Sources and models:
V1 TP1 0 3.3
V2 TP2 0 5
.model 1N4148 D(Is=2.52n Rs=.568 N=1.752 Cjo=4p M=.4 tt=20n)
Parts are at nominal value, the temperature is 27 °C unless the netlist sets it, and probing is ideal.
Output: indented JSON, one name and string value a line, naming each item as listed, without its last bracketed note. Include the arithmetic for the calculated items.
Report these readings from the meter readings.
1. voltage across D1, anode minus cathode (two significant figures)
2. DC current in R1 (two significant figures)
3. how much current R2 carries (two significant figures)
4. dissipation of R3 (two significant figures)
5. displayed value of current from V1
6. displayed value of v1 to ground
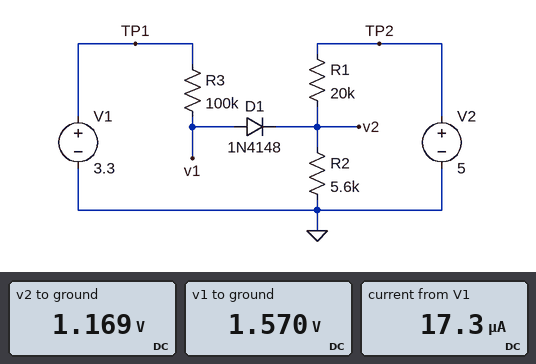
{
  "voltage across D1, anode minus cathode": "1.57 V - 1.169 V = 400 mV",
  "DC current in R1": "(5 V - 1.169 V) / 20 kΩ = 190 µA",
  "how much current R2 carries": "(1.169 V) / 5.6 kΩ = 210 µA",
  "dissipation of R3": "(3.3 V - 1.57 V)^2 / 100 kΩ = 30 µW",
  "displayed value of current from V1": "17.3 µA",
  "displayed value of v1 to ground": "1.570 V"
}
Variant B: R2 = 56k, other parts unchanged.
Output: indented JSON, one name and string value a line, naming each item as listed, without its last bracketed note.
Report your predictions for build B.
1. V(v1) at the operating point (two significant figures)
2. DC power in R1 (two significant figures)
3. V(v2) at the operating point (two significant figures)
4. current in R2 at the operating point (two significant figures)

{
  "V(v1) at the operating point": "3.3 V",
  "DC power in R1": "87 µW",
  "V(v2) at the operating point": "3.7 V",
  "current in R2 at the operating point": "66 µA"
}
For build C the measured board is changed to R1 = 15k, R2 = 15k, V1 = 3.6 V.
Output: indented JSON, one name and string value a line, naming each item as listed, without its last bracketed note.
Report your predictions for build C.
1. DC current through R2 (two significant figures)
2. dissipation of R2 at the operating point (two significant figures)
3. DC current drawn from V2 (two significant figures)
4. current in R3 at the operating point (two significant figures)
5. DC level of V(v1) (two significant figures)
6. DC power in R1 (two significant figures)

{
  "DC current through R2": "170 µA",
  "dissipation of R2 at the operating point": "430 µW",
  "DC current drawn from V2": "160 µA",
  "current in R3 at the operating point": "6.9 µA",
  "DC level of V(v1)": "2.9 V",
  "DC power in R1": "400 µW"
}
